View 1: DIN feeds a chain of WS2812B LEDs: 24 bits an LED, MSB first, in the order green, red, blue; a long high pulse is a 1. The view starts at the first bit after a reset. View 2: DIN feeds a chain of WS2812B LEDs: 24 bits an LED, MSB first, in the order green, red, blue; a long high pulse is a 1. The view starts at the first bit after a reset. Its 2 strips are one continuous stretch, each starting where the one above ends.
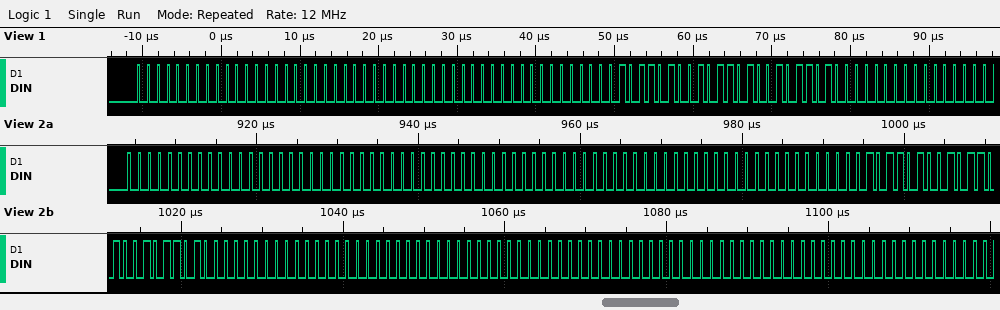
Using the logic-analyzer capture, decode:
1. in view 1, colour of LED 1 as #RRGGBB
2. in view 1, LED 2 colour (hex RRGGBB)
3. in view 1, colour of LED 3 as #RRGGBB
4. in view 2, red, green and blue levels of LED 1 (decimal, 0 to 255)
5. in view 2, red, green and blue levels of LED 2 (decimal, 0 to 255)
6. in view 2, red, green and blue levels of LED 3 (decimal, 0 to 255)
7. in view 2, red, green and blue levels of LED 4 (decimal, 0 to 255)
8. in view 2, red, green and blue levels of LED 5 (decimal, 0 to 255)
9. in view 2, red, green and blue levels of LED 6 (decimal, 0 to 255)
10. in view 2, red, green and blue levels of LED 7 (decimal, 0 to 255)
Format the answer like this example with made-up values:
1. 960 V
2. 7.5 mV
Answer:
1. #000000
2. #000000
3. #5A5A5A
4. 0, 0, 0
5. 0, 0, 0
6. 0, 0, 0
7. 90, 90, 90
8. 0, 0, 0
9. 0, 0, 0
10. 0, 0, 0
